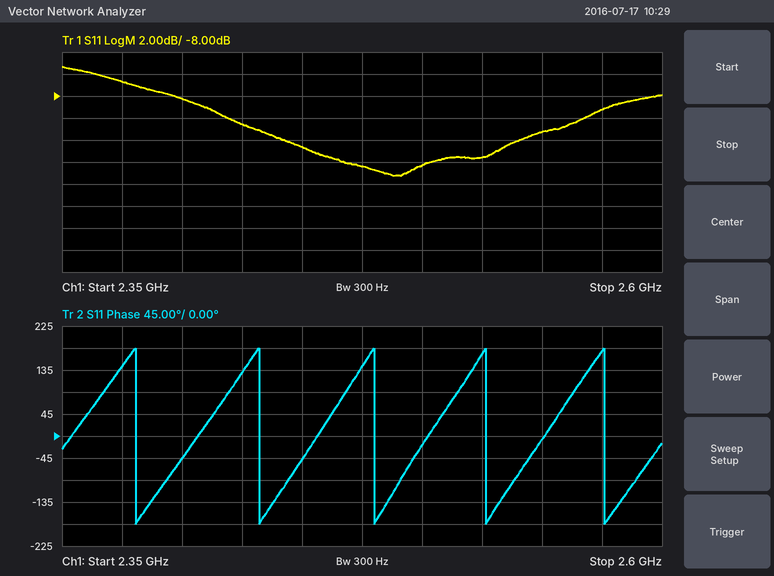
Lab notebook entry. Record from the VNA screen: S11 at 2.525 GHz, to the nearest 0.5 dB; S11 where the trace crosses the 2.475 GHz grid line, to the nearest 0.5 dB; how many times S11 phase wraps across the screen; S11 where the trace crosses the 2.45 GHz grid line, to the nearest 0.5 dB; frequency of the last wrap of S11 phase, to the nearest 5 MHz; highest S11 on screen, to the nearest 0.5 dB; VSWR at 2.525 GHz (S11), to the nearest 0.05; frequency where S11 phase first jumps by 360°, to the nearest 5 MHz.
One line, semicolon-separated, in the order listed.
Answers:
-13.5 dB; -14.5 dB; 5; -12.5 dB; 2.575 GHz; -5.5 dB; 1.55; 2.380 GHz
